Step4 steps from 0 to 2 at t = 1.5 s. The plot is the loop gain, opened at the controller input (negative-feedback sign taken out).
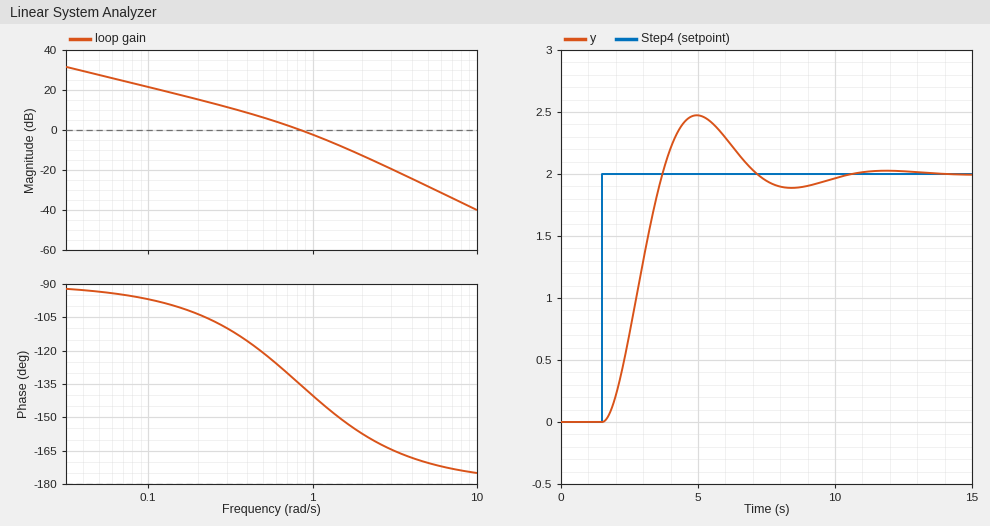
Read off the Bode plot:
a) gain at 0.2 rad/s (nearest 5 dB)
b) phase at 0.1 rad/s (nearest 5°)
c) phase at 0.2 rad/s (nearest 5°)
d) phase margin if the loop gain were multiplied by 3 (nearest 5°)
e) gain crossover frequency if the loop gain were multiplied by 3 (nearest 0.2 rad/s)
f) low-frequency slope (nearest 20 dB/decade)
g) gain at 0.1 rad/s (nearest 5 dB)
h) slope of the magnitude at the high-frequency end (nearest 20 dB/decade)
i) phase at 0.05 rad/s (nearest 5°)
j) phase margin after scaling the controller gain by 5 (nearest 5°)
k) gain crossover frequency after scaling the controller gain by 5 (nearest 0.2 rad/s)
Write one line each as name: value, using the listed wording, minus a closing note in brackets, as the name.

gain at 0.2 rad/s: 15 dB
phase at 0.1 rad/s: -95°
phase at 0.2 rad/s: -105°
phase margin if the loop gain were multiplied by 3: 25°
gain crossover frequency if the loop gain were multiplied by 3: 1.6 rad/s
low-frequency slope: -20 dB/decade
gain at 0.1 rad/s: 20 dB
slope of the magnitude at the high-frequency end: -40 dB/decade
phase at 0.05 rad/s: -95°
phase margin after scaling the controller gain by 5: 20°
gain crossover frequency after scaling the controller gain by 5: 2.2 rad/s
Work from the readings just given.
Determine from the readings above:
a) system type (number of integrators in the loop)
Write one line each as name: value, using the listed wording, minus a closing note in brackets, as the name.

system type: 1
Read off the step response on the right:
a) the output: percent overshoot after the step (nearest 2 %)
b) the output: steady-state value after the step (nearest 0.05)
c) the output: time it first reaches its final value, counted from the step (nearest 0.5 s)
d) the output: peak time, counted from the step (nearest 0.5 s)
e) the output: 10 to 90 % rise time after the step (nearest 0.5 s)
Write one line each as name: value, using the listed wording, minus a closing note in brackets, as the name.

the output: percent overshoot after the step: 24 %
the output: steady-state value after the step: 2.00
the output: time it first reaches its final value, counted from the step: 2.0 s
the output: peak time, counted from the step: 3.5 s
the output: 10 to 90 % rise time after the step: 1.5 s
